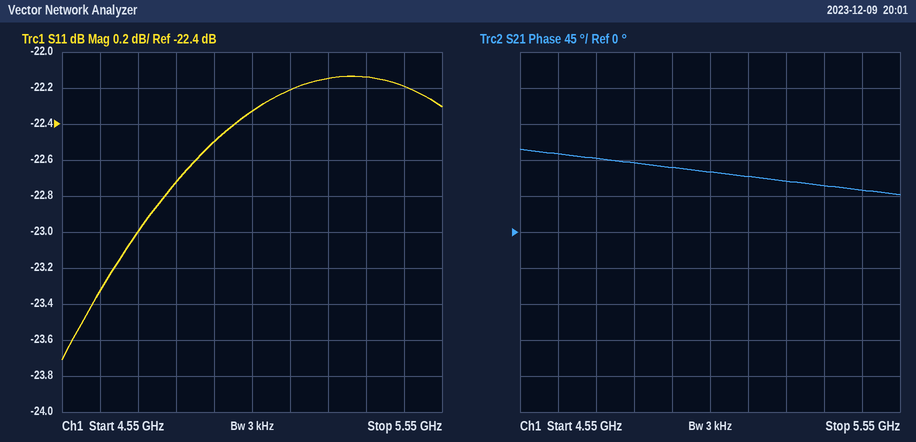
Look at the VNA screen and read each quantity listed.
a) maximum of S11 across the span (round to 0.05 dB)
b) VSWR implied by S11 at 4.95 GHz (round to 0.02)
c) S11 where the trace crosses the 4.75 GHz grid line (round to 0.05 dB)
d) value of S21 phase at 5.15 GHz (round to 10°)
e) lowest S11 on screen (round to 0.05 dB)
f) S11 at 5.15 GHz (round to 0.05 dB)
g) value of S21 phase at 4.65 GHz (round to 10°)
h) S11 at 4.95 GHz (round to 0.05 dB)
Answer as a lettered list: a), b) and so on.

a) -22.15 dB
b) 1.16
c) -23.00 dB
d) 70°
e) -23.70 dB
f) -22.20 dB
g) 100°
h) -22.50 dB
